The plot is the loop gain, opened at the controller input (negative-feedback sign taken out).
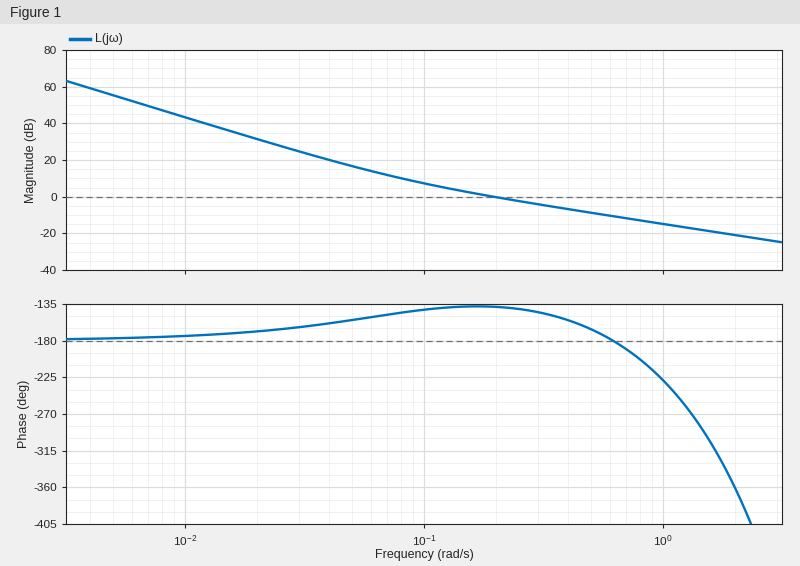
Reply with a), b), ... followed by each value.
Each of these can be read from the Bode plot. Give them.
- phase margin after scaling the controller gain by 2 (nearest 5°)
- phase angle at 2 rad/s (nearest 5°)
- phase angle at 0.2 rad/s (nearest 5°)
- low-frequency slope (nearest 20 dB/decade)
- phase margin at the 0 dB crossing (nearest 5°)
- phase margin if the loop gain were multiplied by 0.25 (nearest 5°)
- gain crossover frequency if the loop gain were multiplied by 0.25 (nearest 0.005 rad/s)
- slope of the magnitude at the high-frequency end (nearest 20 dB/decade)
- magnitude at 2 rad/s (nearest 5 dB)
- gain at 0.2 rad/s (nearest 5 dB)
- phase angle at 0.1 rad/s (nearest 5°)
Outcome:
a) 30°
b) -360°
c) -140°
d) -40 dB/decade
e) 40°
f) 30°
g) 0.070 rad/s
h) -20 dB/decade
i) -20 dB
j) 0 dB
k) -140°
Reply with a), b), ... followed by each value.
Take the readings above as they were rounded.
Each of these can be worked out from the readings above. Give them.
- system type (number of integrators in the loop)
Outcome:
a) 2
